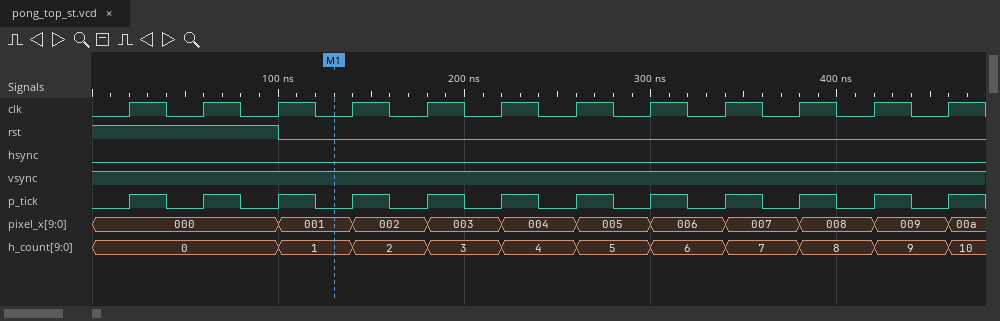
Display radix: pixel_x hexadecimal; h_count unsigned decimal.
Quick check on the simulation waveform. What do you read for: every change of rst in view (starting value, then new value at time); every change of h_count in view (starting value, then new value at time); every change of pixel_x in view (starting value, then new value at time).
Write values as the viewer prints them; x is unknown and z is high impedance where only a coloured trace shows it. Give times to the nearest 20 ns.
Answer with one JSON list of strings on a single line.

["1, 0 at 100 ns", "0, 1 at 100 ns, 2 at 140 ns, 3 at 180 ns, 4 at 220 ns, 5 at 260 ns, 6 at 300 ns, 7 at 340 ns, 8 at 380 ns, 9 at 420 ns, 10 at 460 ns", "000, 001 at 100 ns, 002 at 140 ns, 003 at 180 ns, 004 at 220 ns, 005 at 260 ns, 006 at 300 ns, 007 at 340 ns, 008 at 380 ns, 009 at 420 ns, 00a at 460 ns"]
